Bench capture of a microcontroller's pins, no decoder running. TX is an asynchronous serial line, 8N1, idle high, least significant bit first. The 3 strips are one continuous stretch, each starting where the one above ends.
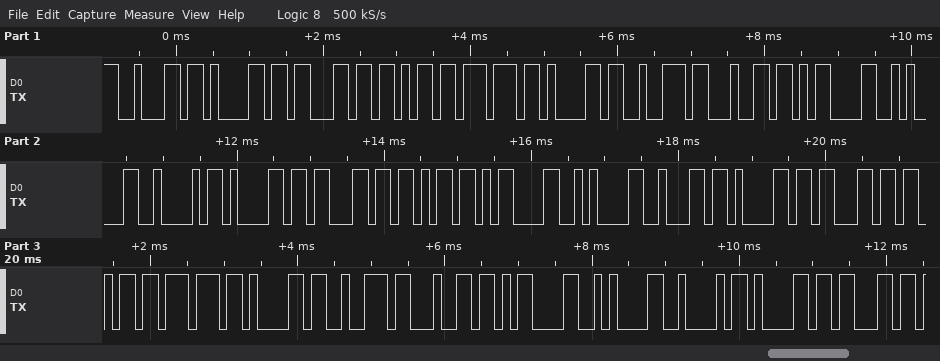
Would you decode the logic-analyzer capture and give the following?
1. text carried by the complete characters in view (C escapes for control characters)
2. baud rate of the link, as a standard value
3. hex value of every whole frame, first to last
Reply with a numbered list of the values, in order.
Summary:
1. "backward\r\nBack\r\nbackward\r\nBac"
2. 9600 baud
3. 62 61 63 6B 77 61 72 64 0D 0A 42 61 63 6B 0D 0A 62 61 63 6B 77 61 72 64 0D 0A 42 61 63
